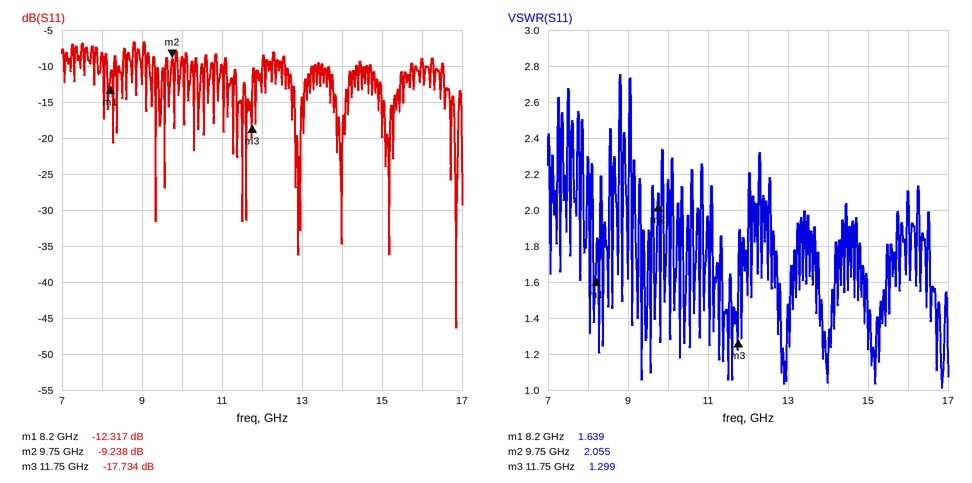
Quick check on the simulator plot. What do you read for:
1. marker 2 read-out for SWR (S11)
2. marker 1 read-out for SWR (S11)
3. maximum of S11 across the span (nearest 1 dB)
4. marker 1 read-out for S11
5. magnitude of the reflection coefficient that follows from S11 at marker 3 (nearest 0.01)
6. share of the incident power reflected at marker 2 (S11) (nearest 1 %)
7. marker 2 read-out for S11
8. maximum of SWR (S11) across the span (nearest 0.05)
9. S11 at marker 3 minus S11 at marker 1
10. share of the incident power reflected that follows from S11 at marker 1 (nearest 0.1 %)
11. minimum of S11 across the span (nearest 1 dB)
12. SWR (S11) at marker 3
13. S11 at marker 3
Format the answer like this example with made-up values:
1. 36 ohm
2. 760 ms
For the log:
1. 2.055
2. 1.639
3. -7 dB
4. -12.317 dB
5. 0.13
6. 12 %
7. -9.238 dB
8. 2.75
9. -5.417 dB
10. 5.9 %
11. -46 dB
12. 1.299
13. -17.734 dB
